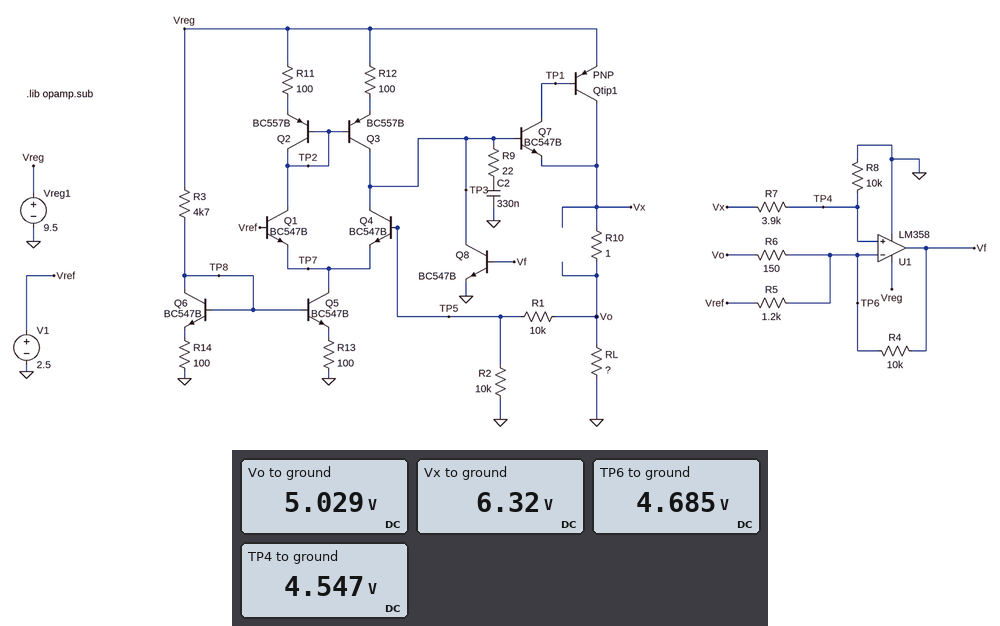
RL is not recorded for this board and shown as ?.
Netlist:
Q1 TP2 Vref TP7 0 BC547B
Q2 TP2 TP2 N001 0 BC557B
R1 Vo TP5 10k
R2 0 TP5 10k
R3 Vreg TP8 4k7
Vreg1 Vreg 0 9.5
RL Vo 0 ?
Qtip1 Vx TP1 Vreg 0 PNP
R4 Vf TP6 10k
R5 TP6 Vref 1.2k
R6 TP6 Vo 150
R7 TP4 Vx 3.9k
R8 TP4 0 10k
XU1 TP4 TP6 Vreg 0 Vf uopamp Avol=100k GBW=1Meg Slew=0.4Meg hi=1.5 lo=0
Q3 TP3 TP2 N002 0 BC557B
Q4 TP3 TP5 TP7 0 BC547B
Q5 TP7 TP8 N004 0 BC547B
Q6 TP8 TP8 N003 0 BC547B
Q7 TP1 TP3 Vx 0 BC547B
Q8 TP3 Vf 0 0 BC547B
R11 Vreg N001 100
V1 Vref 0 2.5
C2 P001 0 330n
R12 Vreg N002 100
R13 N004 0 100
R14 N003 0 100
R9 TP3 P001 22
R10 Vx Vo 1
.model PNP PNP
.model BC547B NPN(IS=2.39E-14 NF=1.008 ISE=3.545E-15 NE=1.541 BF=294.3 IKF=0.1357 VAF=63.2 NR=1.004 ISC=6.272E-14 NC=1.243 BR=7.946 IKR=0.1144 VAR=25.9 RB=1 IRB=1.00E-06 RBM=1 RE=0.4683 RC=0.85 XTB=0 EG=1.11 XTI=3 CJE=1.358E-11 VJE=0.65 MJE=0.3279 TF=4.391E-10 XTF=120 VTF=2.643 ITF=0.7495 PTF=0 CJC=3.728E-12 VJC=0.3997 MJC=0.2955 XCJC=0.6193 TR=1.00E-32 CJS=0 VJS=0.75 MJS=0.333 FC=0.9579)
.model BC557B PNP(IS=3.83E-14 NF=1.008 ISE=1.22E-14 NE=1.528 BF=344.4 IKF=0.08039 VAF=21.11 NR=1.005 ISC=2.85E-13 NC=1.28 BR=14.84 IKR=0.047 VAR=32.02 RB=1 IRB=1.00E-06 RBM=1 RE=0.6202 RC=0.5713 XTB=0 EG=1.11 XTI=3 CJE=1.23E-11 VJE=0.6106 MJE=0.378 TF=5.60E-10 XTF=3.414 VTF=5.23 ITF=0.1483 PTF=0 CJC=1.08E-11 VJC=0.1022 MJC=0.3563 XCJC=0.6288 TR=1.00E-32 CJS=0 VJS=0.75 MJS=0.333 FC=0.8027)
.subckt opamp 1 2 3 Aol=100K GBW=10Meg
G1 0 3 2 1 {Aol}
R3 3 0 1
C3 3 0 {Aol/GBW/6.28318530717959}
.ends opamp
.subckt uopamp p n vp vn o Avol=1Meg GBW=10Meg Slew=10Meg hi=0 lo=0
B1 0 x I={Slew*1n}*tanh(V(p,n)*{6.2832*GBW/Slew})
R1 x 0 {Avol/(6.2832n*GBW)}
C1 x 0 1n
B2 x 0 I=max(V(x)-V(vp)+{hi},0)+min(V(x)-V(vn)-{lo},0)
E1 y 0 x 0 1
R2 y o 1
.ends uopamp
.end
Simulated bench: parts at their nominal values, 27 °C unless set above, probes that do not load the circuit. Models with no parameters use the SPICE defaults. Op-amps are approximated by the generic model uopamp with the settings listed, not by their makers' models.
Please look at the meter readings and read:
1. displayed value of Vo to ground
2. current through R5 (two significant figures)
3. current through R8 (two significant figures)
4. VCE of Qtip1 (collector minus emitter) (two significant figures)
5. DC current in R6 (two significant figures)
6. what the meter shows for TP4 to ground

5.029 V
1.8 mA
450 µA
-3.2 V
2.3 mA
4.547 V
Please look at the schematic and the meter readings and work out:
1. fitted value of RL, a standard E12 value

3.9 Ω
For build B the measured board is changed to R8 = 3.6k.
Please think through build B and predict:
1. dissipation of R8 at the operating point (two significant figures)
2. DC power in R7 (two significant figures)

2.6 mW
2.8 mW
